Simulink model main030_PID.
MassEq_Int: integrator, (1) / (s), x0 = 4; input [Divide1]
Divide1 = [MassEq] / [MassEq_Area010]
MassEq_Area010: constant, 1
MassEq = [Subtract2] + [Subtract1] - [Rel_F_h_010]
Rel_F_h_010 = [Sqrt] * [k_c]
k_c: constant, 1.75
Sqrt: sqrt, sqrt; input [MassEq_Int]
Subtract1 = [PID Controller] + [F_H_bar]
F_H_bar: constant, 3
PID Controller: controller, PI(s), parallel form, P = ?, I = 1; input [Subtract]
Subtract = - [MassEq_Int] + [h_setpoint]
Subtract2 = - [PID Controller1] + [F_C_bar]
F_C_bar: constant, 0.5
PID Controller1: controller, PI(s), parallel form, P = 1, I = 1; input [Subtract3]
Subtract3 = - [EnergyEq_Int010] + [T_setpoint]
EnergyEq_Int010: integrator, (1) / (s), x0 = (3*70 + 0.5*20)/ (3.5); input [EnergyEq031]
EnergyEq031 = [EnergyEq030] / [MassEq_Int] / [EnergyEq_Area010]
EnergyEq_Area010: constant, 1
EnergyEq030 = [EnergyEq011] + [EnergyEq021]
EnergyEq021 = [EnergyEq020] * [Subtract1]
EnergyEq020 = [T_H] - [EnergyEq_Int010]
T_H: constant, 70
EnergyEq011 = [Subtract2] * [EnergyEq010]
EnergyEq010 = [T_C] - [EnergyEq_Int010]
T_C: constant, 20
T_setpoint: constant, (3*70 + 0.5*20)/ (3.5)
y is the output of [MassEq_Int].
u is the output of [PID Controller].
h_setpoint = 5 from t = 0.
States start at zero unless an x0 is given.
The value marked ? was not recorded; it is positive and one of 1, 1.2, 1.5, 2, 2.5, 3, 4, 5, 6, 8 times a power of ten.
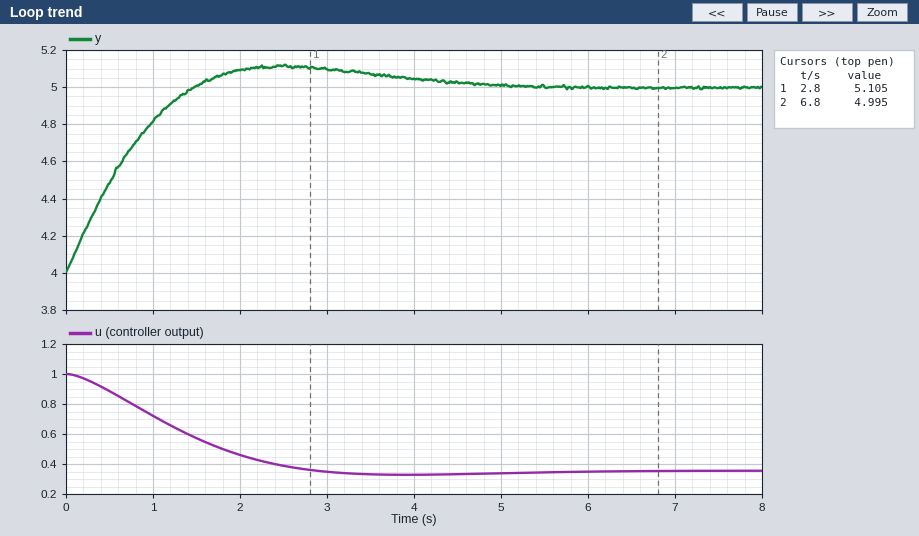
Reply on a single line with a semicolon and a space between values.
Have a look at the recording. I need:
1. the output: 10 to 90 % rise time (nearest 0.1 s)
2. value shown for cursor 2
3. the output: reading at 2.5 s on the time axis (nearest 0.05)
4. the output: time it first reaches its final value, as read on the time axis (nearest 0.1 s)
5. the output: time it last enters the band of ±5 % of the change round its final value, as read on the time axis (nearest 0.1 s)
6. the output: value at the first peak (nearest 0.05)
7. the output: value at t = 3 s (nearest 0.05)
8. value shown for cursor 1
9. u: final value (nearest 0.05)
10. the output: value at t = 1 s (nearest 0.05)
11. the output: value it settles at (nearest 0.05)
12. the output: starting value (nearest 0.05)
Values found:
1.1 s; 4.995; 5.10; 1.5 s; 3.9 s; 5.10; 5.10; 5.105; 0.35; 4.80; 5.00; 4.00
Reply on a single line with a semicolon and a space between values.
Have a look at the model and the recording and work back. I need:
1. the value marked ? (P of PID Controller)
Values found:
1
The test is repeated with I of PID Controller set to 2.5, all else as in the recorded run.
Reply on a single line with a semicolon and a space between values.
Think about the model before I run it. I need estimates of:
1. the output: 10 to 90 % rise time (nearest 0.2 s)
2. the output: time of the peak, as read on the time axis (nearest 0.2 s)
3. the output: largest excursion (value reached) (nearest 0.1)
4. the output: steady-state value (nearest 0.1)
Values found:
0.6 s; 1.6 s; 5.3; 5.0
